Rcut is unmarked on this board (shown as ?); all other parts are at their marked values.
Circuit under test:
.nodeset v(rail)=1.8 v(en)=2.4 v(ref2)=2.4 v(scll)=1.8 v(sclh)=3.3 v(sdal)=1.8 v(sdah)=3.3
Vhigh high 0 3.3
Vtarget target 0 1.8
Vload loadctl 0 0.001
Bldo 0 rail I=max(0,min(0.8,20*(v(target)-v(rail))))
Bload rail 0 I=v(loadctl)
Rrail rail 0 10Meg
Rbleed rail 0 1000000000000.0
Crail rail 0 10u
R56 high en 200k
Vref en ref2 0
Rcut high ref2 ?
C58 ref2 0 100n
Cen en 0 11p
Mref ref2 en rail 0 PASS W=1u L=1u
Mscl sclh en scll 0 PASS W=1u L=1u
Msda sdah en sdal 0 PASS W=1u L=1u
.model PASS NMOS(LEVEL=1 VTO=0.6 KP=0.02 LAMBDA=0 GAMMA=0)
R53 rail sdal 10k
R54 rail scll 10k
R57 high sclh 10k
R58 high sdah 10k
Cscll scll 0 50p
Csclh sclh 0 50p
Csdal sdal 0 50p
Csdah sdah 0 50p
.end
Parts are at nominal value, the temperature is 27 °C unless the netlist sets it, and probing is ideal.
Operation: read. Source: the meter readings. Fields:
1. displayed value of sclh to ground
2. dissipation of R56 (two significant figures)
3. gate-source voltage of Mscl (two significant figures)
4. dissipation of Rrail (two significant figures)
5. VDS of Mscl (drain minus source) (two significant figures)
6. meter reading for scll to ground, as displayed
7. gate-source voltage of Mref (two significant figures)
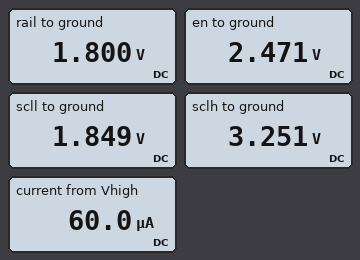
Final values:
3.251 V
3.4 µW
620 mV
320 nW
1.4 V
1.849 V
670 mV
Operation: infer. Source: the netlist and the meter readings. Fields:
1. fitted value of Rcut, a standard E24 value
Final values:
18 kΩ
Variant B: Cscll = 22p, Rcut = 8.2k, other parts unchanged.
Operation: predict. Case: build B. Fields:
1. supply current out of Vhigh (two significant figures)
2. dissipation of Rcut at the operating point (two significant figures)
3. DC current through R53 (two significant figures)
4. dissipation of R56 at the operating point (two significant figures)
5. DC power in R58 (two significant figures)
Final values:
120 µA
78 µW
7.4 µA
3.2 µW
540 nW
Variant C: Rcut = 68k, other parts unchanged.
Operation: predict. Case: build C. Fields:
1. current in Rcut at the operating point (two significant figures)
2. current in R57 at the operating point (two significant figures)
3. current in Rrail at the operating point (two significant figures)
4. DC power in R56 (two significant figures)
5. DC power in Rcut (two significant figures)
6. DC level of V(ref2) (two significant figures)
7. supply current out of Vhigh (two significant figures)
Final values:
13 µA
2.5 µA
180 nA
3.7 µW
11 µW
2.4 V
22 µA
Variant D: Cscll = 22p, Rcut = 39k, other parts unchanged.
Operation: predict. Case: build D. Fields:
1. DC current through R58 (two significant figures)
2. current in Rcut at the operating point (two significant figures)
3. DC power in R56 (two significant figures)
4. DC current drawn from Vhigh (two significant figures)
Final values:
3.3 µA
22 µA
3.6 µW
33 µA
